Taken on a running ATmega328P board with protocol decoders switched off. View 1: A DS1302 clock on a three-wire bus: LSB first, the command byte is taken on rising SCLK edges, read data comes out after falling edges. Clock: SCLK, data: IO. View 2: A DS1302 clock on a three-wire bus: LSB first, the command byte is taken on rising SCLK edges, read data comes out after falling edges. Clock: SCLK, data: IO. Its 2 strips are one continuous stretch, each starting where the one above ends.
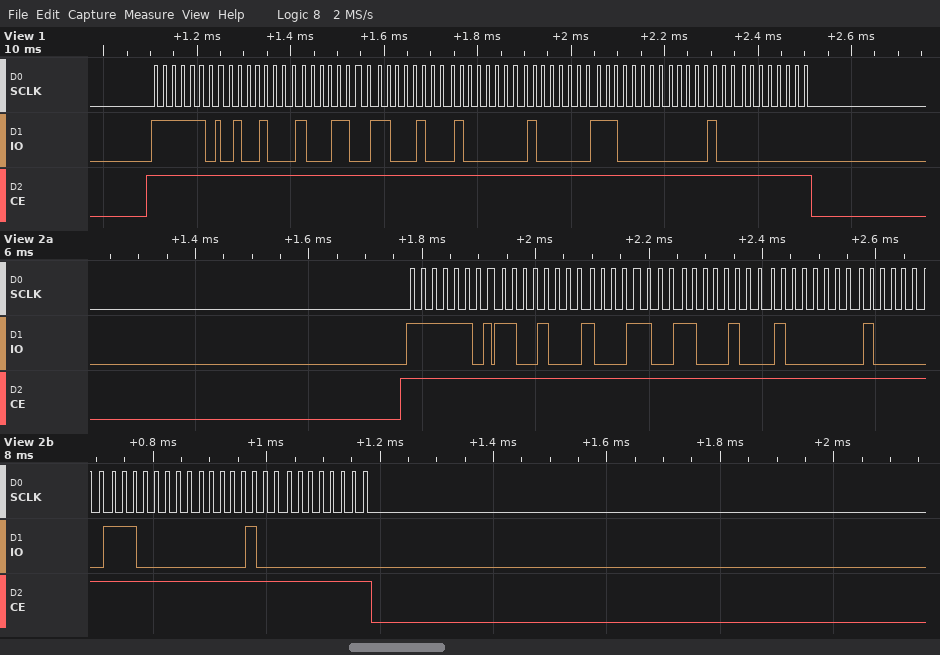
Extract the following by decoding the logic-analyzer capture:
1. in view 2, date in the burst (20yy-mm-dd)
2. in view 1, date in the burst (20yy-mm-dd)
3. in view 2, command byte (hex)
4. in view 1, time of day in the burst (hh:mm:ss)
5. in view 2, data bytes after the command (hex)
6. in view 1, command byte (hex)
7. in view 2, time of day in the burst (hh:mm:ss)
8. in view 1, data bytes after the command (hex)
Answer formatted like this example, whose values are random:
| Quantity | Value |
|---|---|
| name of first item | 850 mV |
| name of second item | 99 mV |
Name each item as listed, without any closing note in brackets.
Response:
| Quantity | Value |
|---|---|
| in view 2, date in the burst | 2020-02-02 |
| in view 1, date in the burst | 2020-02-02 |
| in view 2, command byte | 0xBF |
| in view 1, time of day in the burst | 23:31:12 |
| in view 2, data bytes after the command | 13 31 23 02 02 07 20 00 |
| in view 1, command byte | 0xBF |
| in view 2, time of day in the burst | 23:31:13 |
| in view 1, data bytes after the command | 12 31 23 02 02 07 20 00 |
